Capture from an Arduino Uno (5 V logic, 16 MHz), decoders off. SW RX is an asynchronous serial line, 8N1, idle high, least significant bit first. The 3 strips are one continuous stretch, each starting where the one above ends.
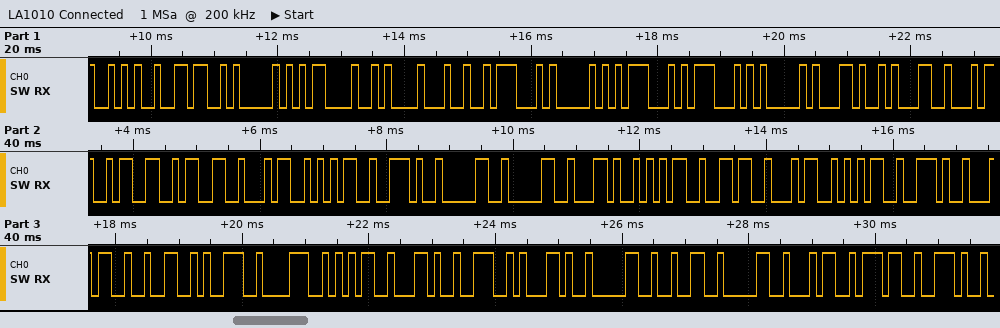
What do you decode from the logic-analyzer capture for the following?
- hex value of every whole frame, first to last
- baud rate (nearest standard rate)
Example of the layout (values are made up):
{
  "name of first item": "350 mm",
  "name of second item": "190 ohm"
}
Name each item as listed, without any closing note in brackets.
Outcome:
{
  "hex value of every whole frame, first to last": "2A 36 41 0D 0A 24 47 50 47 47 41 2C 31 34 33 33 34 35 2E 30 30 2C 35 36 34 35 2E 34 32 39 38 35 2C 4E 2C 30 32 30 34 37 2E",
  "baud rate": "9600 baud"
}
